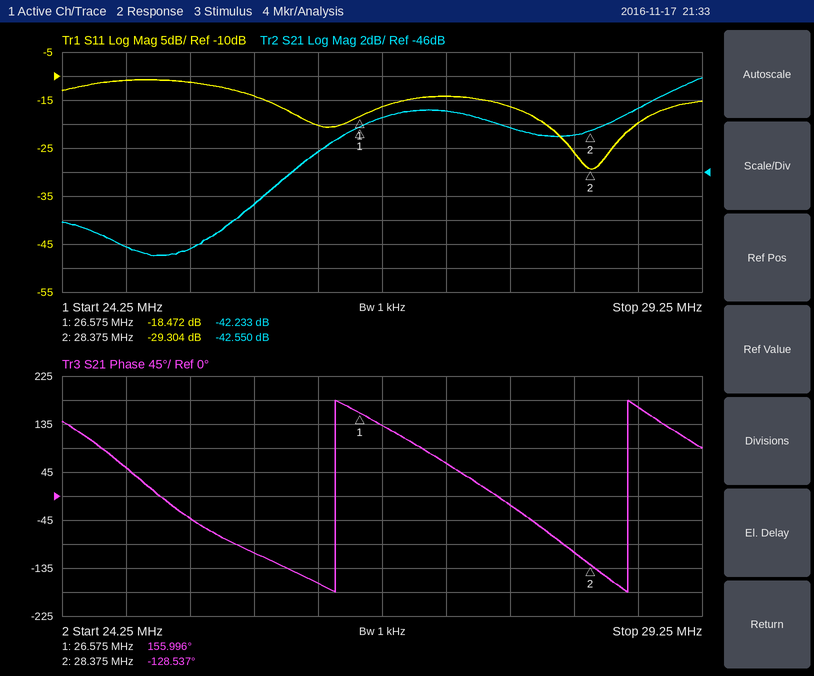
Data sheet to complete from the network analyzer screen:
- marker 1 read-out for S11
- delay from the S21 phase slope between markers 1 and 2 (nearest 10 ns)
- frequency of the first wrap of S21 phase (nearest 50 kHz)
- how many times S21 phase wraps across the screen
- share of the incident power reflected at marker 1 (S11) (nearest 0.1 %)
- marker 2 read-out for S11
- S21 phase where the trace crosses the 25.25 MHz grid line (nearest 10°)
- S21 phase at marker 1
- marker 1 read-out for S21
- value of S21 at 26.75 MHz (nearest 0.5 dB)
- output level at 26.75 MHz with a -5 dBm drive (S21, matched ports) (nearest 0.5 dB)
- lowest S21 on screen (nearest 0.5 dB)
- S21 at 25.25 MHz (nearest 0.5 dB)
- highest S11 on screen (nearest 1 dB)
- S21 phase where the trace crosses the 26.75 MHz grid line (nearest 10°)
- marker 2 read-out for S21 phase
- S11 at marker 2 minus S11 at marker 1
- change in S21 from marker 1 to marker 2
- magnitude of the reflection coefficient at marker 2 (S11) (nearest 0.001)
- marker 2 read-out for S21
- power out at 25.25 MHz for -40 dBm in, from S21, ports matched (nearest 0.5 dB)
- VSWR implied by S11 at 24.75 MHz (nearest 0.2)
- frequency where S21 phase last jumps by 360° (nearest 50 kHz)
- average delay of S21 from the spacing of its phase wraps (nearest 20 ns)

-18.472 dB
440 ns
26.40 MHz
2
1.4 %
-29.304 dB
-40°
155.996°
-42.233 dB
-41.5 dB
-46.5 dBm
-53.0 dB
-52.5 dB
-11 dB
130°
-128.537°
-10.832 dB
-0.317 dB
0.034
-42.550 dB
-92.5 dBm
1.8
28.65 MHz
440 ns
